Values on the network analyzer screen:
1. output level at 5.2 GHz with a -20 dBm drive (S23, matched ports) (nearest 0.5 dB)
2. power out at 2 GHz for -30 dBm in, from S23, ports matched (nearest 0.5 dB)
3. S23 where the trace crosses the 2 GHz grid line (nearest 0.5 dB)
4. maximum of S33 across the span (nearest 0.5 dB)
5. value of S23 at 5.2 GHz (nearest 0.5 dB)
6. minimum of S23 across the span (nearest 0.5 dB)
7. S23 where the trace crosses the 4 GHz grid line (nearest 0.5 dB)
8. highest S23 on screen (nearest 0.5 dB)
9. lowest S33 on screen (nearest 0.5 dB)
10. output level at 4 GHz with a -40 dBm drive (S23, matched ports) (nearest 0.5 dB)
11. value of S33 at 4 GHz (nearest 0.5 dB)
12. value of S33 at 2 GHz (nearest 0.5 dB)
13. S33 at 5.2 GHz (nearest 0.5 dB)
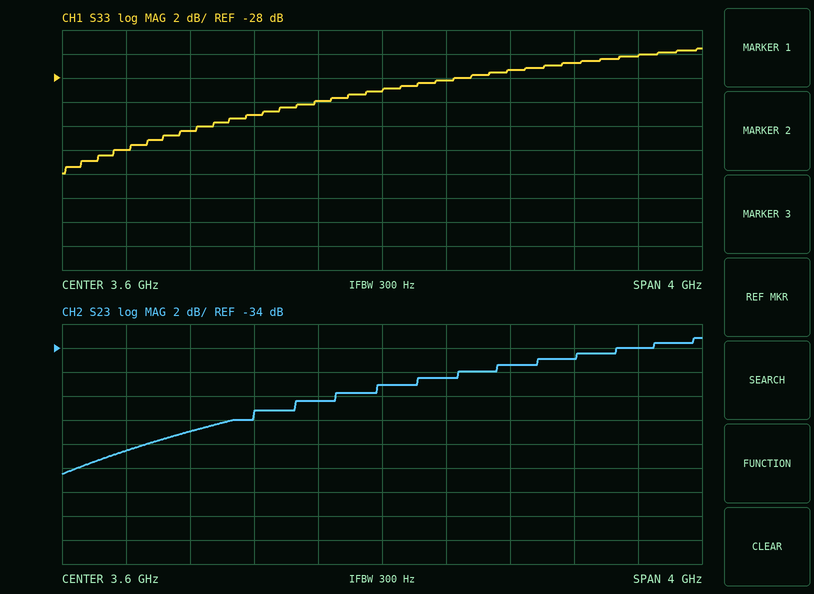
-54.0 dBm
-72.5 dBm
-42.5 dB
-25.5 dB
-34.0 dB
-44.5 dB
-36.5 dB
-33.0 dB
-36.0 dB
-76.5 dBm
-28.0 dB
-34.0 dB
-26.0 dB
